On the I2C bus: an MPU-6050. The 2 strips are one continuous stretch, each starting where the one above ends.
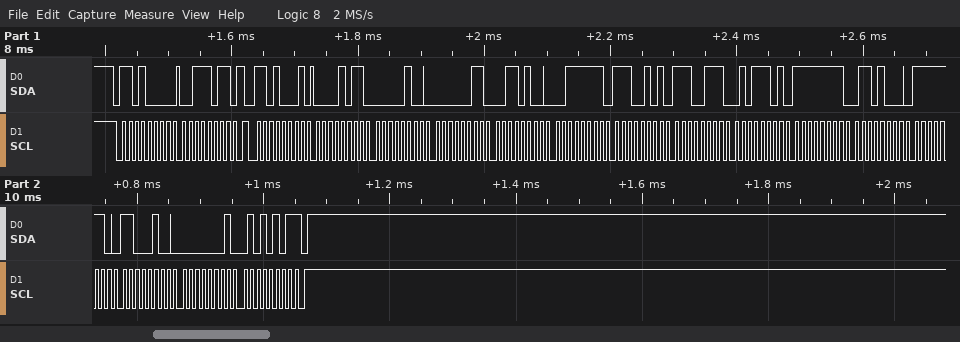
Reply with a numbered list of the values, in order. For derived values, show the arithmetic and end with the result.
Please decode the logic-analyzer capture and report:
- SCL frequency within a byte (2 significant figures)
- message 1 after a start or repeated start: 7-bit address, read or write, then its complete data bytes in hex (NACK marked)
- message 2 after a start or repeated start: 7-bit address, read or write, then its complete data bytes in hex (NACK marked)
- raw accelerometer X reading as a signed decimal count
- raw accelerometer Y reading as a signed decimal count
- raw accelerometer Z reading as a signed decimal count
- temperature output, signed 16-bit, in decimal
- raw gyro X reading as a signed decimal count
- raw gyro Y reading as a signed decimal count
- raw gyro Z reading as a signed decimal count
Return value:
1. 100 kHz
2. 0x68 write: 3B
3. 0x68 read: 0B 04 03 34 3F E5 E7 5D FF 68 FE C4 01 55 NACK
4. 0x0B04 = 2820
5. 0x0334 = 820
6. 0x3FE5 = 16357
7. 0xE75D = -6307
8. 0xFF68 = -152
9. 0xFEC4 = -316
10. 0x0155 = 341
